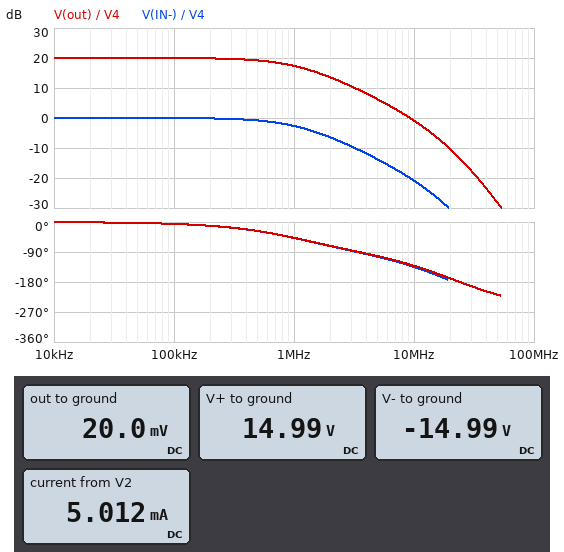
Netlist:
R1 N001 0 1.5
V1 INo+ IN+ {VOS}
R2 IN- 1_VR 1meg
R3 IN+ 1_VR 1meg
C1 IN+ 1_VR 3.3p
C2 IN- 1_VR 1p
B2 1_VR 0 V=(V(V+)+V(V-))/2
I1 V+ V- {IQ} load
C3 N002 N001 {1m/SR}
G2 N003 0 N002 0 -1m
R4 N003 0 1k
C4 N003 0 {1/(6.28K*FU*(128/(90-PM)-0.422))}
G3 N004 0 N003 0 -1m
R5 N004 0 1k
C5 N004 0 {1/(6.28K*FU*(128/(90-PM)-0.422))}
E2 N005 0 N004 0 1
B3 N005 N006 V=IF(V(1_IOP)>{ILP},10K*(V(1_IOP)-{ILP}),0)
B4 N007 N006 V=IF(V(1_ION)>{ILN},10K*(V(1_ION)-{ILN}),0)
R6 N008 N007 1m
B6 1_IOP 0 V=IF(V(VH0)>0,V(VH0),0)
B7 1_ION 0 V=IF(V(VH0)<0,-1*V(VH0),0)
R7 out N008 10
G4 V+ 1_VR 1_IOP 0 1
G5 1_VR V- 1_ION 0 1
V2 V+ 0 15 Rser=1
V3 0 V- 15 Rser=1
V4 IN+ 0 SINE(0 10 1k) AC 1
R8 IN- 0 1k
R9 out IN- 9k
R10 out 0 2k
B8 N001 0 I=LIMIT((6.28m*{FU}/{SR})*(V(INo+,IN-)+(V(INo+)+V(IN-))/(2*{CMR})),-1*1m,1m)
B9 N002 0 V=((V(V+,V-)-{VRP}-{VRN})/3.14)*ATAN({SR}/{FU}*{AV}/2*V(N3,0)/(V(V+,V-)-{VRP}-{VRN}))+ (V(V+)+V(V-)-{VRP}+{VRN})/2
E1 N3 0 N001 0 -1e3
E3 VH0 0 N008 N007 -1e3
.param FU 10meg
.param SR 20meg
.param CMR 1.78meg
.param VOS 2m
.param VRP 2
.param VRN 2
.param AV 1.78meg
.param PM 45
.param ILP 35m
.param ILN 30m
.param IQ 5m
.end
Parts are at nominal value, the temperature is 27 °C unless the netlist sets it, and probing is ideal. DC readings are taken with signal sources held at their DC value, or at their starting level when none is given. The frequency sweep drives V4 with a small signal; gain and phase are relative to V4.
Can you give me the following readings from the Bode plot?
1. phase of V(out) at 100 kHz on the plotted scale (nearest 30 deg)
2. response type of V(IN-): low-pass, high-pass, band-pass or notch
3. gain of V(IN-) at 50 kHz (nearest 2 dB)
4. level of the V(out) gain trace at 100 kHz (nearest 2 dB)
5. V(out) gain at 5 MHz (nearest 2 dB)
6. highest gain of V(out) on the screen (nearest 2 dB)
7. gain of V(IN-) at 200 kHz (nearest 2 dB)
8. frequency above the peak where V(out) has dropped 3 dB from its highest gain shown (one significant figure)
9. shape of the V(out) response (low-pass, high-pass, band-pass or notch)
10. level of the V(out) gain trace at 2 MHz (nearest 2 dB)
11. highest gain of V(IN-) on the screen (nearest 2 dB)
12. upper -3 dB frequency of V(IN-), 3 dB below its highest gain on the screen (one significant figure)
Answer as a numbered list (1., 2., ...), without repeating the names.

1. 0 deg
2. low-pass
3. 0 dB
4. 20 dB
5. 6 dB
6. 20 dB
7. 0 dB
8. 1 MHz
9. low-pass
10. 14 dB
11. 0 dB
12. 1 MHz
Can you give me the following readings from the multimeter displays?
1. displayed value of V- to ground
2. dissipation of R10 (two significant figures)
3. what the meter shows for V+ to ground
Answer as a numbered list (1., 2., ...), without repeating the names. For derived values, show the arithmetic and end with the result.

1. -14.99 V
2. (20 mV)^2 / 2 kΩ = 200 nW
3. 14.99 V
